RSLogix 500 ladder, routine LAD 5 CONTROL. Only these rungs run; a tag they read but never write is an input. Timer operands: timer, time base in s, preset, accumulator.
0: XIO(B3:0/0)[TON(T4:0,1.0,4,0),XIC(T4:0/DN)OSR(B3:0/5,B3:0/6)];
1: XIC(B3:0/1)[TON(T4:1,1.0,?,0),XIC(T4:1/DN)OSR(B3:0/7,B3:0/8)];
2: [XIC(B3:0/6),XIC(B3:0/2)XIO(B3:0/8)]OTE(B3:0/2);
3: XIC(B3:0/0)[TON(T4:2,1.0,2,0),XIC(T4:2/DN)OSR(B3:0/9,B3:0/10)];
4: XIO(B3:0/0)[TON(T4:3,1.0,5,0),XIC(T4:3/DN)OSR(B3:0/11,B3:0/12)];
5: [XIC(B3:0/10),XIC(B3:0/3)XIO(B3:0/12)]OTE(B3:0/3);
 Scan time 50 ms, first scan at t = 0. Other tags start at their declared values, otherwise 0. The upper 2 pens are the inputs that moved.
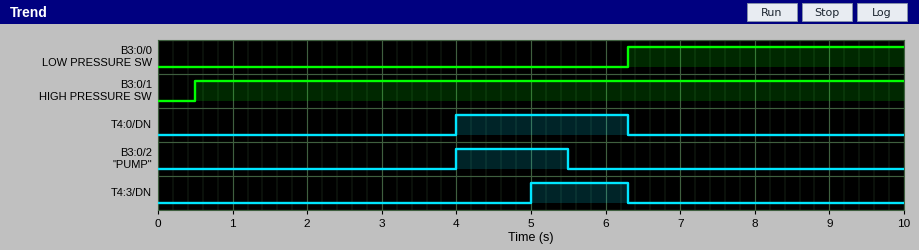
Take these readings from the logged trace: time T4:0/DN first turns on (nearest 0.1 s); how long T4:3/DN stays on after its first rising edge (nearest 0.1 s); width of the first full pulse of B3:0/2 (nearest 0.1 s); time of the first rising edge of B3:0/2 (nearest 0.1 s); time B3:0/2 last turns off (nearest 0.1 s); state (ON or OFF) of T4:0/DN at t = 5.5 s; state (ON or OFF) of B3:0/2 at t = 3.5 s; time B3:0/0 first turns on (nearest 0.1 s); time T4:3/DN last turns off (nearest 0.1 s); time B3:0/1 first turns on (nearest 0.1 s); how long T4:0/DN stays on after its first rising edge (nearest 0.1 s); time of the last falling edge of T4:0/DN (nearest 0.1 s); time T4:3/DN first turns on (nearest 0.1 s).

4.0 s
1.3 s
1.5 s
4.0 s
5.5 s
ON
OFF
6.3 s
6.3 s
0.5 s
2.3 s
6.3 s
5.0 s
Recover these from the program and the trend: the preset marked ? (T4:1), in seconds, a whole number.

5 s
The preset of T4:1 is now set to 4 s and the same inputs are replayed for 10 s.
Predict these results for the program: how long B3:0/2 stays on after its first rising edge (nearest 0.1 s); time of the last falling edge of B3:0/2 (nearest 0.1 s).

0.5 s
4.5 s
